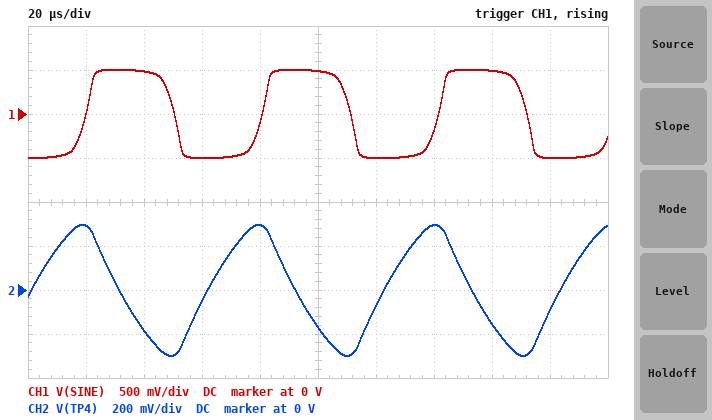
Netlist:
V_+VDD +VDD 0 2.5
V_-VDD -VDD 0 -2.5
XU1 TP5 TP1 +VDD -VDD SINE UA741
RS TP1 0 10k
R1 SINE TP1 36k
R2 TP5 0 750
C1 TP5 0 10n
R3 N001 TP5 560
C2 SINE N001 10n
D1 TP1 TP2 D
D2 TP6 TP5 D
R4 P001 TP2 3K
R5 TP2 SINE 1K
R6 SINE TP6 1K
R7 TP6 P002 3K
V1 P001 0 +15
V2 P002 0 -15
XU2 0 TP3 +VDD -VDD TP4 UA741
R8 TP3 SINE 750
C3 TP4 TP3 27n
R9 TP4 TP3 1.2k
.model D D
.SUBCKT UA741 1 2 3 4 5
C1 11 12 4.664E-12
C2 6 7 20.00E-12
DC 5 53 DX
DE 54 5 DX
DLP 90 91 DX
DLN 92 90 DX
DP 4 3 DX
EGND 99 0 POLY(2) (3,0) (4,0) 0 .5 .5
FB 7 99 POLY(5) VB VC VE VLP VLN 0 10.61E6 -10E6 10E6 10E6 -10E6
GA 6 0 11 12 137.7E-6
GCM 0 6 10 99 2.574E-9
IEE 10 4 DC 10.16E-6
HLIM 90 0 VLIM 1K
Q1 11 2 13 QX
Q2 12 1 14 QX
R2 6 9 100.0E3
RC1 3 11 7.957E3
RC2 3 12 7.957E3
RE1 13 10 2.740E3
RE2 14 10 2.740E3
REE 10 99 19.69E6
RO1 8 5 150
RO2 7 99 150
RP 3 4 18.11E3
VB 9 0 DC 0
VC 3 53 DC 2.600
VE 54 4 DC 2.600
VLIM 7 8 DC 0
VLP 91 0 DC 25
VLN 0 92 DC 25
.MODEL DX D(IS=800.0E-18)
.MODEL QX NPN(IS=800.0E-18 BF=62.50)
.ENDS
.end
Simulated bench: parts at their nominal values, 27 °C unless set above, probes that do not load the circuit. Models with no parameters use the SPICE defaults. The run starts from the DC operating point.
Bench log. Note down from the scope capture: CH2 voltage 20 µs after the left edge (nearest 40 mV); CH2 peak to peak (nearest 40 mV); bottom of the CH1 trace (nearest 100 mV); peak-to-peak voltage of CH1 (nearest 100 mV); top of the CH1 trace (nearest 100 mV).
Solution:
280 mV
600 mV
-500 mV
1.0 V
500 mV
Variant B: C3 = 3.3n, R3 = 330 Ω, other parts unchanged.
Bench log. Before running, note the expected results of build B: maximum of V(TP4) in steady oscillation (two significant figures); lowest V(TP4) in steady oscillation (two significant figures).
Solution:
500 mV
-500 mV
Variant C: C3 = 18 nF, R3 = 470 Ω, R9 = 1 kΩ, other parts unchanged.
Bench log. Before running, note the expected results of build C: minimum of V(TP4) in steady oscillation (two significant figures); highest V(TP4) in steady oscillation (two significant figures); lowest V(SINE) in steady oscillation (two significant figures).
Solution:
-390 mV
390 mV
-500 mV
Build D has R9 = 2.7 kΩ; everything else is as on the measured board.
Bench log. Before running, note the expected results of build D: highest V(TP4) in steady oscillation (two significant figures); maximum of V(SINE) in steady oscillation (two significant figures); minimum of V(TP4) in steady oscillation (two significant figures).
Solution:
310 mV
500 mV
-320 mV
